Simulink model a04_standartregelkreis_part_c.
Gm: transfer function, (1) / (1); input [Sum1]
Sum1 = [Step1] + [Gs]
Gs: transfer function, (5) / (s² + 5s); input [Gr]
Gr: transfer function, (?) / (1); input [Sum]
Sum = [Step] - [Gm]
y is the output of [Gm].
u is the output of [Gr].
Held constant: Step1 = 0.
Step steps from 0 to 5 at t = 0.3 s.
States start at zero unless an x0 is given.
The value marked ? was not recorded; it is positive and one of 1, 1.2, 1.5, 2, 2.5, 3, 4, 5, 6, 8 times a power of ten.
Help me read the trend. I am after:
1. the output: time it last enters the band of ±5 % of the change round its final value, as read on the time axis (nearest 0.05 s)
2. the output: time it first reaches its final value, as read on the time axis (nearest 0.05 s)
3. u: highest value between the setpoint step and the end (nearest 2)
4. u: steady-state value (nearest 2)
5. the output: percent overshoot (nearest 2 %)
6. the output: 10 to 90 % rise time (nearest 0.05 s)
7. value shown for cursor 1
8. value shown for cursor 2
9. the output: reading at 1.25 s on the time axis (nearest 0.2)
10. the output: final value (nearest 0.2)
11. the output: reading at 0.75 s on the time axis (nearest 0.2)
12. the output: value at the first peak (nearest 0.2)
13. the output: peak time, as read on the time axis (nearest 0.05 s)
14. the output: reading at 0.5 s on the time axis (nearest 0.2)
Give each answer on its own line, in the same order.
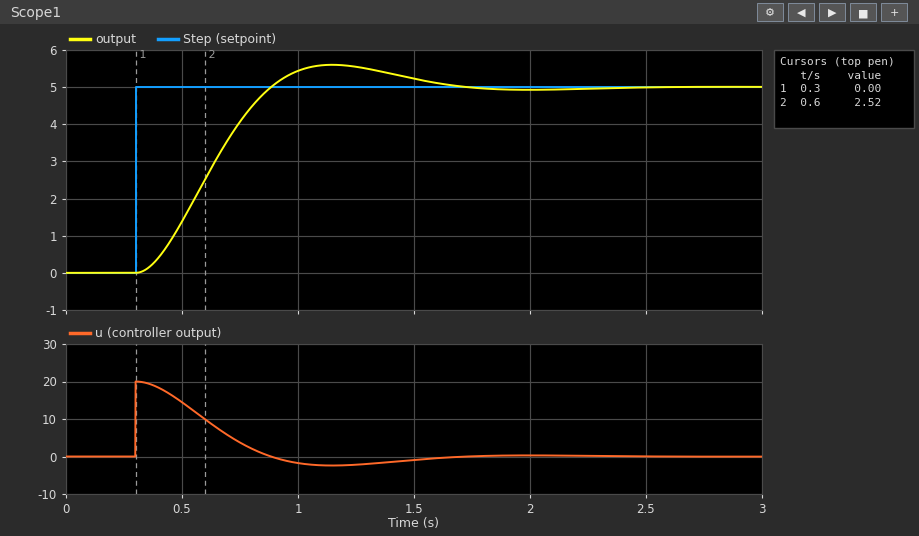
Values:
1.50 s
0.90 s
20
0
12 %
0.40 s
0.00
2.52
5.6
5.0
4.0
5.6
1.15 s
1.4
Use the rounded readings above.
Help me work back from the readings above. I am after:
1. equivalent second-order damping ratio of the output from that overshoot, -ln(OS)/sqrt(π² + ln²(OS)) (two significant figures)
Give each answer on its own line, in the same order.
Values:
0.56
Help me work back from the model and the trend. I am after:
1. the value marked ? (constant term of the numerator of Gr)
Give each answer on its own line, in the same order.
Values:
4
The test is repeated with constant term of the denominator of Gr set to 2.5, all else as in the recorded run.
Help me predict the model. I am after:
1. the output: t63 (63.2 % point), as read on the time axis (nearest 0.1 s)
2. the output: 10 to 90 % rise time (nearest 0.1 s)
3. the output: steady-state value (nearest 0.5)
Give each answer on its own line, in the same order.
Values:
1.0 s
1.0 s
5.0
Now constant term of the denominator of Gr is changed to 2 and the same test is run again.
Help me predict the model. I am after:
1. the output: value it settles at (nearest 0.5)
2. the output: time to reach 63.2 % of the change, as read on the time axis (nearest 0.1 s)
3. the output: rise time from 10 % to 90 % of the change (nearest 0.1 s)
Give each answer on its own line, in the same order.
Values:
5.0
0.9 s
0.8 s
